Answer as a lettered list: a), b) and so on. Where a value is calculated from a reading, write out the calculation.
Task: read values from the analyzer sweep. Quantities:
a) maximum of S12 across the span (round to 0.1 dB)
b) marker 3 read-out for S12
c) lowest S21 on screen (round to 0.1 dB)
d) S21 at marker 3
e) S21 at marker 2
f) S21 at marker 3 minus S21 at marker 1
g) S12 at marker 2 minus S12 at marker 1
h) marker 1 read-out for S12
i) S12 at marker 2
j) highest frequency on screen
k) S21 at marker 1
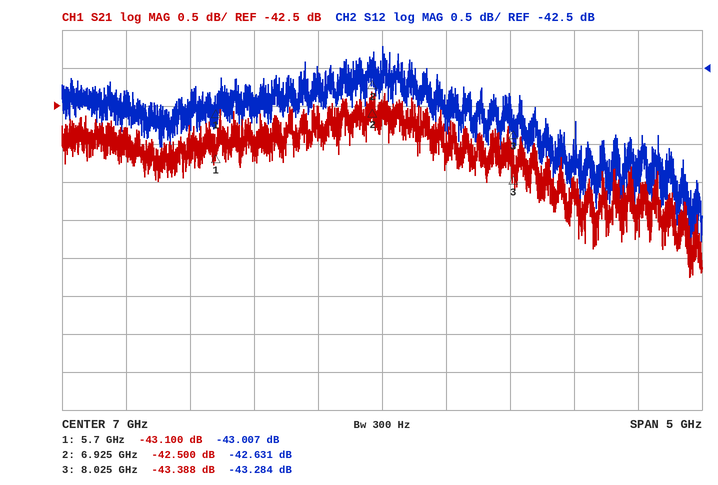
a) -42.2 dB
b) -43.284 dB
c) -44.8 dB
d) -43.388 dB
e) -42.500 dB
f) -43.388 − (-43.1) = -0.288 dB
g) -42.631 − (-43.007) = 0.376 dB
h) -43.007 dB
i) -42.631 dB
j) 9.5 GHz
k) -43.100 dB
